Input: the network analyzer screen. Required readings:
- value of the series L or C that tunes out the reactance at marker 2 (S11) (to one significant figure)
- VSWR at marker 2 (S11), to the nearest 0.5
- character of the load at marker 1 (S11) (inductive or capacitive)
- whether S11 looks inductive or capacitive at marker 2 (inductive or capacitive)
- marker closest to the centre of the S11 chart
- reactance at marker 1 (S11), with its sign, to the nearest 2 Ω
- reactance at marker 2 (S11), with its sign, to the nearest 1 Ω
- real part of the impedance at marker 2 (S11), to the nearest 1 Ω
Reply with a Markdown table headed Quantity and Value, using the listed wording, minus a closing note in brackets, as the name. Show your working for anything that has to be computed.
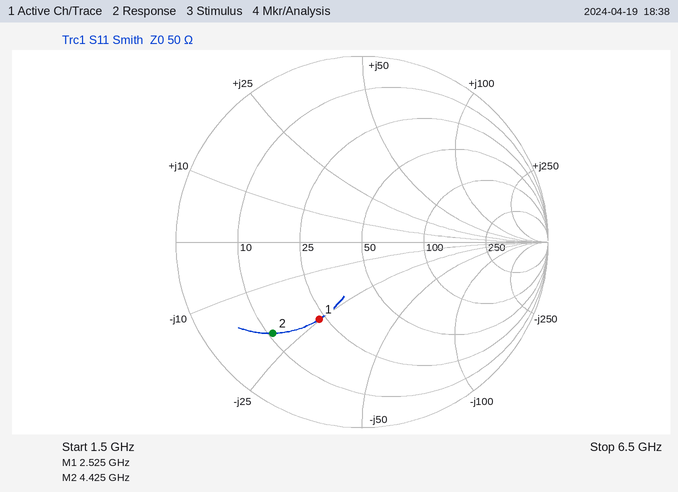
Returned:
| Quantity | Value |
|---|---|
| value of the series L or C that tunes out the reactance at marker 2 (S11) | L = 20 Ω/(2π × 4.425 GHz) ≈ 719 pH, so 700 pH to one significant figure |
| VSWR at marker 2 (S11), to the nearest 0.5 | 5.5 |
| character of the load at marker 1 (S11) | capacitive |
| whether S11 looks inductive or capacitive at marker 2 | capacitive |
| marker closest to the centre of the S11 chart | marker 1 |
| reactance at marker 1 (S11), with its sign, to the nearest 2 Ω | -24 Ω |
| reactance at marker 2 (S11), with its sign, to the nearest 1 Ω | -20 Ω |
| real part of the impedance at marker 2 (S11), to the nearest 1 Ω | 11 Ω |
